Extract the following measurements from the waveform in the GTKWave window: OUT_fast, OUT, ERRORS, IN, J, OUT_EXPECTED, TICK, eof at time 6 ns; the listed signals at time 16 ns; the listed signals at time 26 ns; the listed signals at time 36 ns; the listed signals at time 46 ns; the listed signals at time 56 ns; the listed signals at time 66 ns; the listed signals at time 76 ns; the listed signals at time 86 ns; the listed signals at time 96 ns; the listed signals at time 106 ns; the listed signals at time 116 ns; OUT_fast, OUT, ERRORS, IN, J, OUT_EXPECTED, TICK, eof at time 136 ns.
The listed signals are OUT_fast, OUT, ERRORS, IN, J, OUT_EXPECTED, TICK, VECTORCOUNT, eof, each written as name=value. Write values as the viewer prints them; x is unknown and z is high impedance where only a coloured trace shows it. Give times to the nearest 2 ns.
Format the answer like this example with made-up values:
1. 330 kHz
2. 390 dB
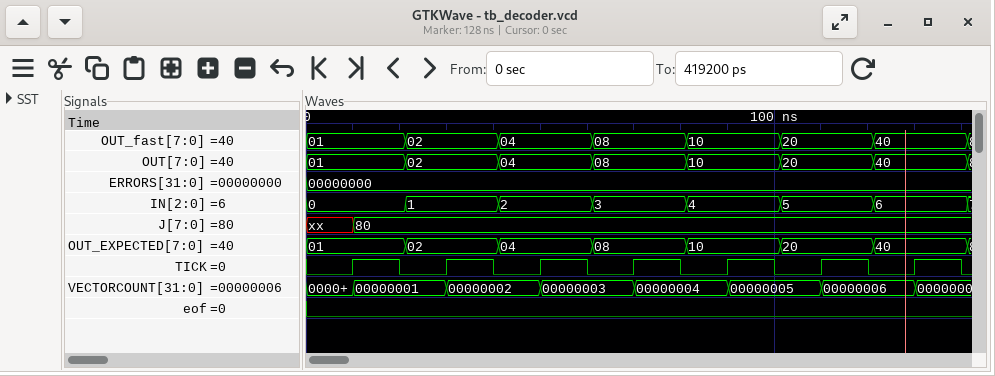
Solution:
1. OUT_fast=01, OUT=01, ERRORS=00000000, IN=0, J=xx, OUT_EXPECTED=01, TICK=0, eof=0
2. OUT_fast=01, OUT=01, ERRORS=00000000, IN=0, J=80, OUT_EXPECTED=01, TICK=1, VECTORCOUNT=00000001, eof=0
3. OUT_fast=02, OUT=02, ERRORS=00000000, IN=1, J=80, OUT_EXPECTED=02, TICK=0, VECTORCOUNT=00000001, eof=0
4. OUT_fast=02, OUT=02, ERRORS=00000000, IN=1, J=80, OUT_EXPECTED=02, TICK=1, VECTORCOUNT=00000002, eof=0
5. OUT_fast=04, OUT=04, ERRORS=00000000, IN=2, J=80, OUT_EXPECTED=04, TICK=0, VECTORCOUNT=00000002, eof=0
6. OUT_fast=04, OUT=04, ERRORS=00000000, IN=2, J=80, OUT_EXPECTED=04, TICK=1, VECTORCOUNT=00000003, eof=0
7. OUT_fast=08, OUT=08, ERRORS=00000000, IN=3, J=80, OUT_EXPECTED=08, TICK=0, VECTORCOUNT=00000003, eof=0
8. OUT_fast=08, OUT=08, ERRORS=00000000, IN=3, J=80, OUT_EXPECTED=08, TICK=1, VECTORCOUNT=00000004, eof=0
9. OUT_fast=10, OUT=10, ERRORS=00000000, IN=4, J=80, OUT_EXPECTED=10, TICK=0, VECTORCOUNT=00000004, eof=0
10. OUT_fast=10, OUT=10, ERRORS=00000000, IN=4, J=80, OUT_EXPECTED=10, TICK=1, VECTORCOUNT=00000005, eof=0
11. OUT_fast=20, OUT=20, ERRORS=00000000, IN=5, J=80, OUT_EXPECTED=20, TICK=0, VECTORCOUNT=00000005, eof=0
12. OUT_fast=20, OUT=20, ERRORS=00000000, IN=5, J=80, OUT_EXPECTED=20, TICK=1, VECTORCOUNT=00000006, eof=0
13. OUT_fast=40, OUT=40, ERRORS=00000000, IN=6, J=80, OUT_EXPECTED=40, TICK=1, eof=0
